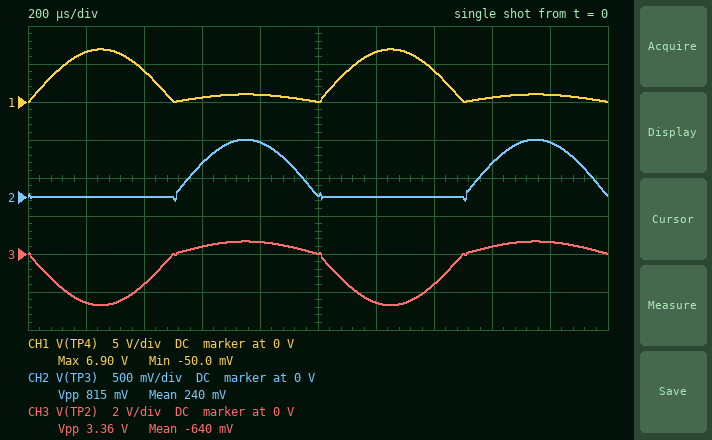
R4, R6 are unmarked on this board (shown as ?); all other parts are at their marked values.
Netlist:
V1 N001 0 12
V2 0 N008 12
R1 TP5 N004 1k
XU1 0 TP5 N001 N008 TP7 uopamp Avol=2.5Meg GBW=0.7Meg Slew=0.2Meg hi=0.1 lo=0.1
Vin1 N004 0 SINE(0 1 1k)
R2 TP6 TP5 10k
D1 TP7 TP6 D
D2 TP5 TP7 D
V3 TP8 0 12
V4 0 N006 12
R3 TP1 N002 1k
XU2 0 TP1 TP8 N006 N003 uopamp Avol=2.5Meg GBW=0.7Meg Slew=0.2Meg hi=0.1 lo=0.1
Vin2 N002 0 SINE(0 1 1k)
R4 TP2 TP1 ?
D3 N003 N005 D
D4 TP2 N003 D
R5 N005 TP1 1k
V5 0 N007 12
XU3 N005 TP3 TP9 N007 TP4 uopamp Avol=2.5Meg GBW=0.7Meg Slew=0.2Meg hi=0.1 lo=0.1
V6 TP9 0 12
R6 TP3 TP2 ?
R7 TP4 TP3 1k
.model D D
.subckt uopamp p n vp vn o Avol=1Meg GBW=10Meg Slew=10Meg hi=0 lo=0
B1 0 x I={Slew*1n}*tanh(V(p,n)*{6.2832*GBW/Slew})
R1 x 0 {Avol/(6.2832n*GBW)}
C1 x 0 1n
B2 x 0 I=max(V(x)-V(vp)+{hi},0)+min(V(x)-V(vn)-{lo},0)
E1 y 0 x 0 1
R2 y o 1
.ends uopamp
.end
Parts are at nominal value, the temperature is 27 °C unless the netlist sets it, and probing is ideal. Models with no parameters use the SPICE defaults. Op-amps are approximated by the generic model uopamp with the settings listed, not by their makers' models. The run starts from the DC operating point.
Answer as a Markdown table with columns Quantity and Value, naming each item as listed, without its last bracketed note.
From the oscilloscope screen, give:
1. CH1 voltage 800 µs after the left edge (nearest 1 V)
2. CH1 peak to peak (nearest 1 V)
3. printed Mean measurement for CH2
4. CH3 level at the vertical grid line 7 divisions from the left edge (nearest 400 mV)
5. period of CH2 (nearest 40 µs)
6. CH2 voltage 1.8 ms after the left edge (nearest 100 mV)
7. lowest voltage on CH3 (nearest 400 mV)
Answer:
| Quantity | Value |
|---|---|
| CH1 voltage 800 µs after the left edge | 1 V |
| CH1 peak to peak | 7 V |
| printed Mean measurement for CH2 | 240 mV |
| CH3 level at the vertical grid line 7 divisions from the left edge | -1.6 V |
| period of CH2 | 1.00 ms |
| CH2 voltage 1.8 ms after the left edge | 700 mV |
| lowest voltage on CH3 | -2.8 V |
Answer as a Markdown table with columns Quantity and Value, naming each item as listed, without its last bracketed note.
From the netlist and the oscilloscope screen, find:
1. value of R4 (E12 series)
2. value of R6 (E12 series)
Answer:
| Quantity | Value |
|---|---|
| value of R4 | 2.7 kΩ |
| value of R6 | 390 Ω |
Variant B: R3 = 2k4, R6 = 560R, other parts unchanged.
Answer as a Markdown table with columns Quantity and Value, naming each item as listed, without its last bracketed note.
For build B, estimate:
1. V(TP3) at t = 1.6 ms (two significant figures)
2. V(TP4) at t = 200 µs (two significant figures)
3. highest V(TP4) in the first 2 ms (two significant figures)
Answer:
| Quantity | Value |
|---|---|
| V(TP3) at t = 1.6 ms | 190 mV |
| V(TP4) at t = 200 µs | 1.9 V |
| highest V(TP4) in the first 2 ms | 2.0 V |
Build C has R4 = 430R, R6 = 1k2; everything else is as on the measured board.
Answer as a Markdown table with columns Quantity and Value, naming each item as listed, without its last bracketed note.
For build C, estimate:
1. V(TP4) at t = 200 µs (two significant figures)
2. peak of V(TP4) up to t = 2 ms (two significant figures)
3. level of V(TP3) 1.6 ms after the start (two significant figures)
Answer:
| Quantity | Value |
|---|---|
| V(TP4) at t = 200 µs | 340 mV |
| peak of V(TP4) up to t = 2 ms | 1.0 V |
| level of V(TP3) 1.6 ms after the start | 360 mV |
